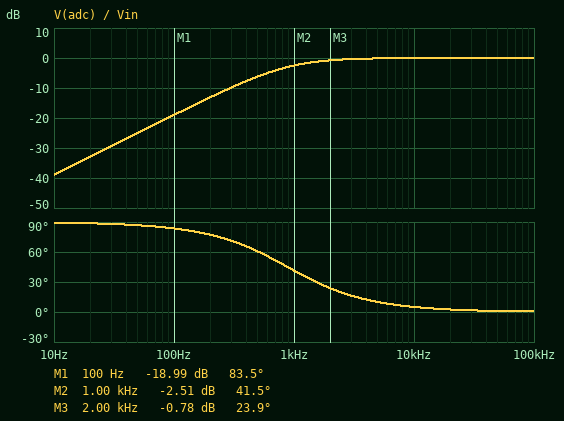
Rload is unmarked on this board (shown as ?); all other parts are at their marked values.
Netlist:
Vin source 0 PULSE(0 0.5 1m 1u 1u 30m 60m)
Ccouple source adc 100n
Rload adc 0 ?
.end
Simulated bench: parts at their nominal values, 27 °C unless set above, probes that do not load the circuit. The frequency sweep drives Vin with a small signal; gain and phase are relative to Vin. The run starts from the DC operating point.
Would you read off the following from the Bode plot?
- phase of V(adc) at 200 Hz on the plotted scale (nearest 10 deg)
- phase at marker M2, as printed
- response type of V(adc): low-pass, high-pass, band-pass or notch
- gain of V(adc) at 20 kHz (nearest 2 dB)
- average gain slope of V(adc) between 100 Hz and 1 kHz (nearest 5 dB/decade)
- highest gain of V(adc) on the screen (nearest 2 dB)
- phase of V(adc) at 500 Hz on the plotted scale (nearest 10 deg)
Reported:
80 deg
41.5 deg
high-pass
0 dB
15 dB/decade
0 dB
60 deg
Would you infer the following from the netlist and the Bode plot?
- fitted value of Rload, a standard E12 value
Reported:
1.8 kΩ
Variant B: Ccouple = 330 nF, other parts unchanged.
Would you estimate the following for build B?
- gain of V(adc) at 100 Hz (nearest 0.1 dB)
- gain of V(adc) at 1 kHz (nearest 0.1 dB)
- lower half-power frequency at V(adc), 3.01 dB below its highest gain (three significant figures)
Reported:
-9.1 dB
-0.3 dB
268 Hz
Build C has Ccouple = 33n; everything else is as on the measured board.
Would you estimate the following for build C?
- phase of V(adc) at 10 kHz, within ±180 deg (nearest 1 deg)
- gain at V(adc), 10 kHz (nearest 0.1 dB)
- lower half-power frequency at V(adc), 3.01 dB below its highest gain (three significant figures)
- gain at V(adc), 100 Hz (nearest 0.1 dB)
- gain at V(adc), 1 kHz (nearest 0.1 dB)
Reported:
15 deg
-0.3 dB
2.68 kHz
-28.6 dB
-9.1 dB
